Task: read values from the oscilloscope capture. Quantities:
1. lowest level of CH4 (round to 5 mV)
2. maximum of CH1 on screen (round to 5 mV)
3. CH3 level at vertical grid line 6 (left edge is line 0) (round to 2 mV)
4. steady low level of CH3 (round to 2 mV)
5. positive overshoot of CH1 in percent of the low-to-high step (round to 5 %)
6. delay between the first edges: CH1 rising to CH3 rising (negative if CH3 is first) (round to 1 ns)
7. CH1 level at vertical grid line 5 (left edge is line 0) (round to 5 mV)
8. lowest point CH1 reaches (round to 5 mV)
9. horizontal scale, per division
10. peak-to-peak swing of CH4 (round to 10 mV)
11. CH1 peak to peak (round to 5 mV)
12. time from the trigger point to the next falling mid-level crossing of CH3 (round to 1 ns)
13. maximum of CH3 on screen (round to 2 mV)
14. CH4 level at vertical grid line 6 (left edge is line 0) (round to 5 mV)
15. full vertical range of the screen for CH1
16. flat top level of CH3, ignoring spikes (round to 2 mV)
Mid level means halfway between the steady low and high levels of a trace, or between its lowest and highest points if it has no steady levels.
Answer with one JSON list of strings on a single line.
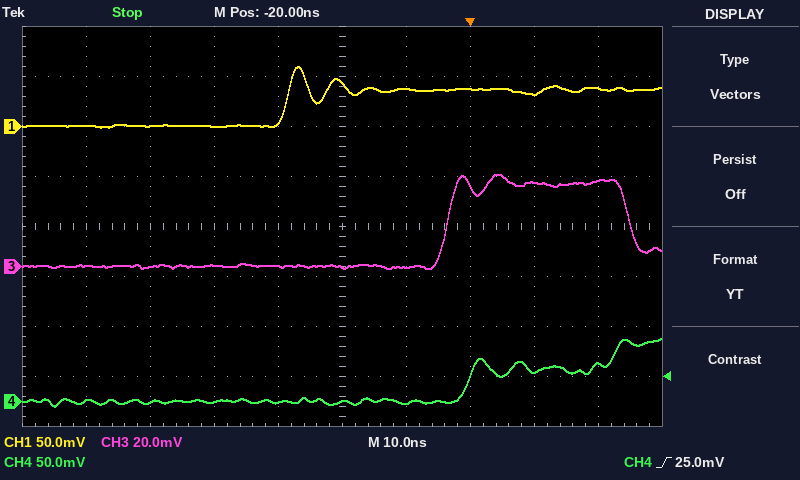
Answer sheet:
["-5 mV", "60 mV", "0 mV", "0 mV", "65 %", "+25 ns", "45 mV", "0 mV", "10 ns", "70 mV", "60 mV", "25 ns", "36 mV", "0 mV", "400 mV", "34 mV"]
